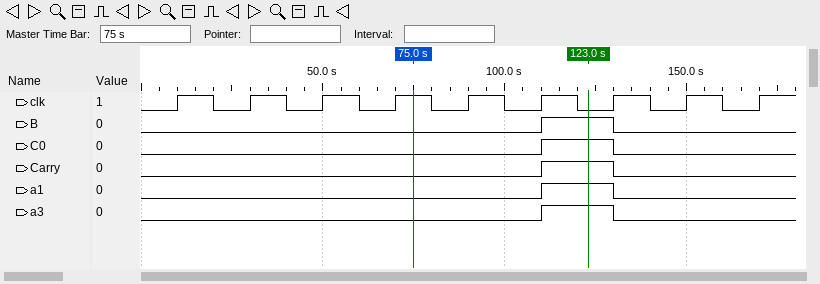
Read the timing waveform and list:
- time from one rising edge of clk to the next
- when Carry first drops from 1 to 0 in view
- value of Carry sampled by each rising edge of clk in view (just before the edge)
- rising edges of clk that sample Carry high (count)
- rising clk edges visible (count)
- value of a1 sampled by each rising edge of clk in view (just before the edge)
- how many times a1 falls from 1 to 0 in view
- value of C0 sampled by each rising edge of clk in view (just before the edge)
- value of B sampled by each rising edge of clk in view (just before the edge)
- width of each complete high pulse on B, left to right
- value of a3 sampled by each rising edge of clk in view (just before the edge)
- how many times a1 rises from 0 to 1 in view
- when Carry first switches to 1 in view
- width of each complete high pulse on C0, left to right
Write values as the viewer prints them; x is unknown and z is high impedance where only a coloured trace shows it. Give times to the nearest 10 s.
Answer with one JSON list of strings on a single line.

["20 s", "130 s", "0 0 0 0 0 0 1 0 0", "1", "9", "0 0 0 0 0 0 1 0 0", "1", "0 0 0 0 0 0 1 0 0", "0 0 0 0 0 0 1 0 0", "20 s", "0 0 0 0 0 0 1 0 0", "1", "110 s", "20 s"]
